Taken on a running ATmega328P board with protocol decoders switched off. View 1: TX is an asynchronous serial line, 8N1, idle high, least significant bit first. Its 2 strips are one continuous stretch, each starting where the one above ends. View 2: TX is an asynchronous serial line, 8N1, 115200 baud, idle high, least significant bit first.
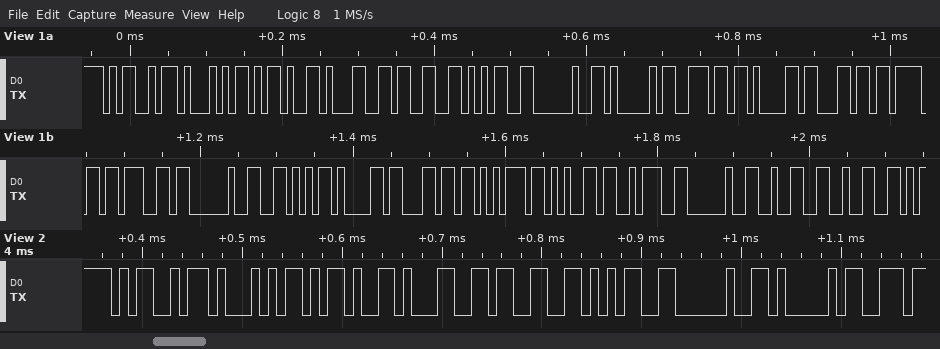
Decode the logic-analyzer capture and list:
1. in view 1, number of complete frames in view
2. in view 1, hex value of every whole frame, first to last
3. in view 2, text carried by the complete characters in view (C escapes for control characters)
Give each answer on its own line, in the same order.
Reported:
23
4D 51 2D 31 33 35 20 41 6E 61 6C 6F 67 20 56 61 6C 75 65 3A 20 32 32
"MQ-135 A"
